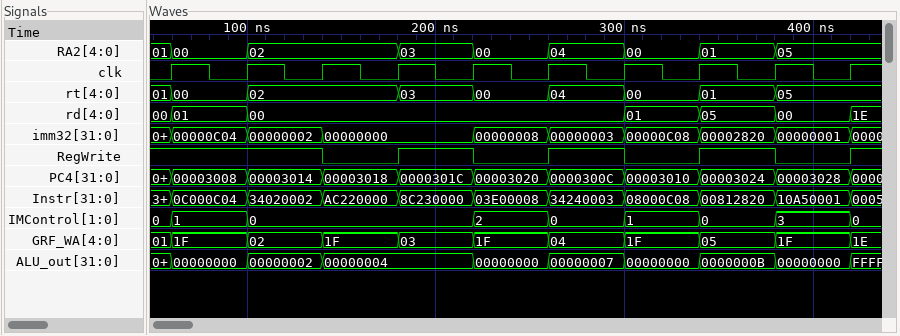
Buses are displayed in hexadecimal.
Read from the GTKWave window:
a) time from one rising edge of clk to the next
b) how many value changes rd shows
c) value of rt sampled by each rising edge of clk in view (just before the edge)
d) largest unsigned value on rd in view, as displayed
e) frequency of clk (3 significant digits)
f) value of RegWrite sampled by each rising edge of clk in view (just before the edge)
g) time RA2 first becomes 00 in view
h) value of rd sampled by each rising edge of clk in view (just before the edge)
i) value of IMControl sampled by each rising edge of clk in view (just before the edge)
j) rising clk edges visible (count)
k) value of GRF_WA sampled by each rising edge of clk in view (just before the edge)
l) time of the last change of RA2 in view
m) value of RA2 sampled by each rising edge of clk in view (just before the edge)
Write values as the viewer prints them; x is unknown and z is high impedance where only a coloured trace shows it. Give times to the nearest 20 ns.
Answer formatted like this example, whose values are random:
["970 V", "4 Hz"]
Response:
["40 ns", "6", "01, 00, 02, 02, 03, 00, 04, 00, 01, 05", "1E", "25.0 MHz", "1 1 1 0 1 0 1 0 1 0", "60 ns", "00, 01, 00, 00, 00, 00, 00, 01, 05, 00", "0, 1, 0, 0, 0, 2, 0, 1, 0, 3", "10", "01, 1F, 02, 1F, 03, 1F, 04, 1F, 05, 1F", "380 ns", "01, 00, 02, 02, 03, 00, 04, 00, 01, 05"]
